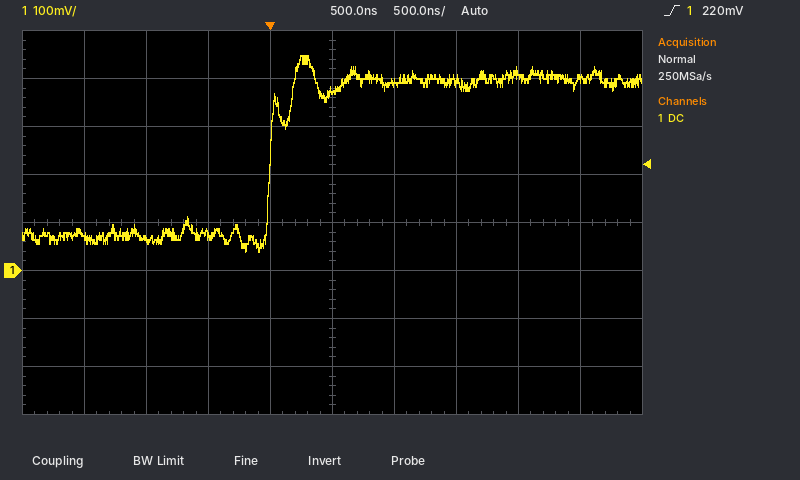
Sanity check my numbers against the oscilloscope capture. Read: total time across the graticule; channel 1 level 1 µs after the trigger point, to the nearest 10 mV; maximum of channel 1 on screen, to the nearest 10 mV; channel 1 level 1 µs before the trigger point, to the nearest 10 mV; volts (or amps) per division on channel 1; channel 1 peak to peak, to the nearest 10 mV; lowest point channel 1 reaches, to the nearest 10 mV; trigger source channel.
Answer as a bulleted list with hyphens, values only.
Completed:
- 5 µs
- 390 mV
- 450 mV
- 60 mV
- 100 mV
- 410 mV
- 40 mV
- channel 1
